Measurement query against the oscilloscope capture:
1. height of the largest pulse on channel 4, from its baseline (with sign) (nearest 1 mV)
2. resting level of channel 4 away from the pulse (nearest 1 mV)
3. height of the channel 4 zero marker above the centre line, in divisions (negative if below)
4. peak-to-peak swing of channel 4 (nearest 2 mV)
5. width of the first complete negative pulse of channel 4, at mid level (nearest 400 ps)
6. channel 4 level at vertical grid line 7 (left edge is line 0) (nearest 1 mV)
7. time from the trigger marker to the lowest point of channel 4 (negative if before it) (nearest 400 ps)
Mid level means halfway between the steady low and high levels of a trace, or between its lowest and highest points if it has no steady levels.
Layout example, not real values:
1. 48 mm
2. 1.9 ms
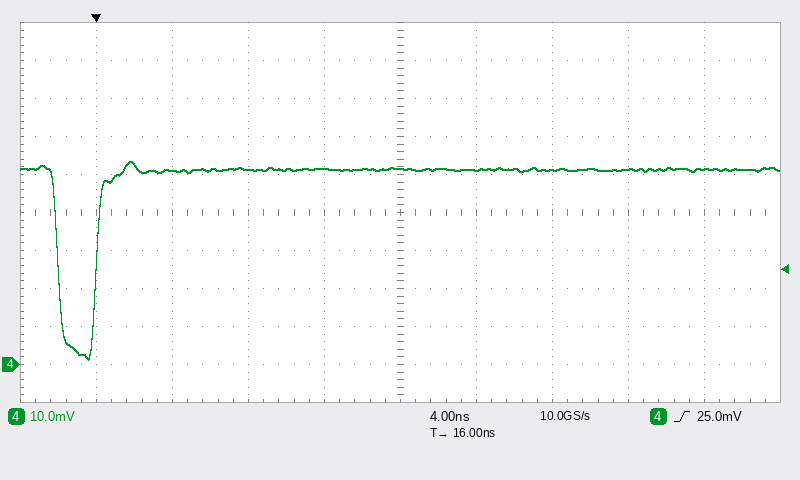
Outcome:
1. -50 mV
2. 51 mV
3. -4.0 div
4. 52 mV
5. 2.0 ns
6. 51 mV
7. -400 ps
